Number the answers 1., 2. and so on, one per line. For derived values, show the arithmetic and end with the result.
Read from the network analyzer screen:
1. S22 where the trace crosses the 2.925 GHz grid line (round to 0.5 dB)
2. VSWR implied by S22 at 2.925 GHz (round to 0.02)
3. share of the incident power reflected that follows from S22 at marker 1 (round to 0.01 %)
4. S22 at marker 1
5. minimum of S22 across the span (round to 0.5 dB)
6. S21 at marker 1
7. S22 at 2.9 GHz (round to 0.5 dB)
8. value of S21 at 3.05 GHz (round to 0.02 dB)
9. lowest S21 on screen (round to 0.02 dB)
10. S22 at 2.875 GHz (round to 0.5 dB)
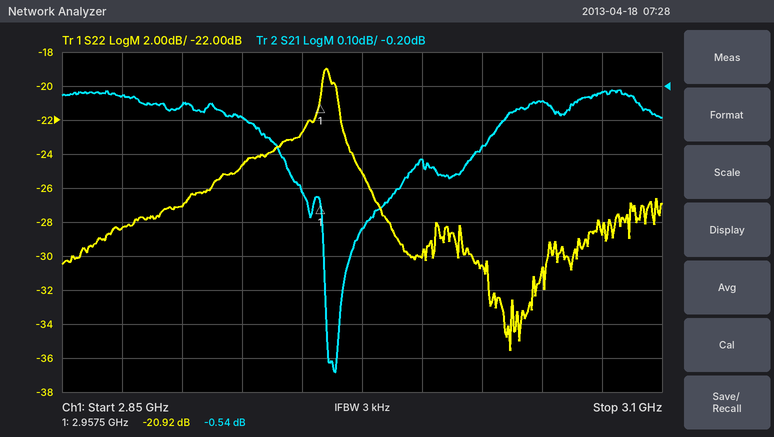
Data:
1. -24.5 dB
2. |Γ| = 10^(-24.5/20) = 0.0596; VSWR = (1 + 0.0596)/(1 − 0.0596) ≈ 1.13, so 1.12 to the nearest 0.02
3. 10^(-20.92/10) ≈ 0.81 %
4. -20.92 dB
5. -35.5 dB
6. -0.54 dB
7. -27.0 dB
8. -0.24 dB
9. -1.04 dB
10. -28.5 dB
